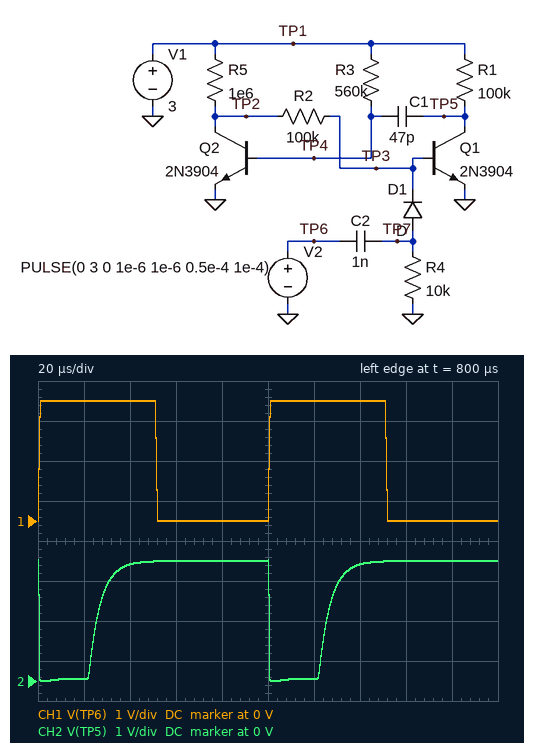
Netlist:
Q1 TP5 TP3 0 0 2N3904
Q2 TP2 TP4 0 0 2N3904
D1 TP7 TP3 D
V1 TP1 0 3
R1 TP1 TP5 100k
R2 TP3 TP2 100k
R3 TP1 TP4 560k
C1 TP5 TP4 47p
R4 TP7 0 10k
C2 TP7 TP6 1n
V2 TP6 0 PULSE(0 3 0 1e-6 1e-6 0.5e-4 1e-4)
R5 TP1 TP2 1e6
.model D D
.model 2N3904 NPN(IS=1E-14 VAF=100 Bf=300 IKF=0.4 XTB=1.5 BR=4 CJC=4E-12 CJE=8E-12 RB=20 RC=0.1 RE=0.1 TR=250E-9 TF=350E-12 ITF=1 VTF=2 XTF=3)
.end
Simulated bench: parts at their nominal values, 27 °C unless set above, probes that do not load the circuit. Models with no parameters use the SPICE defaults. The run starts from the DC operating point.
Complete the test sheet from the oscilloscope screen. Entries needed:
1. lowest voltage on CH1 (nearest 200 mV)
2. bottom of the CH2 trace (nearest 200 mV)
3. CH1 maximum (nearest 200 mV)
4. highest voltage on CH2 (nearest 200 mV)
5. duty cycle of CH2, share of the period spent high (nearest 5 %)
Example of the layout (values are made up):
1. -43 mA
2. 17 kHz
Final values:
1. 0 V
2. 0 V
3. 3.0 V
4. 3.0 V
5. 75 %
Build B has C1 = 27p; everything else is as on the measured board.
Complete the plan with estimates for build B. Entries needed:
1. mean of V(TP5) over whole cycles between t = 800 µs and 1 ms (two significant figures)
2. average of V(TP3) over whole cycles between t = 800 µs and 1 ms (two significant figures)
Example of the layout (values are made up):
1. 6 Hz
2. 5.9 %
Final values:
1. 2.5 V
2. 100 mV
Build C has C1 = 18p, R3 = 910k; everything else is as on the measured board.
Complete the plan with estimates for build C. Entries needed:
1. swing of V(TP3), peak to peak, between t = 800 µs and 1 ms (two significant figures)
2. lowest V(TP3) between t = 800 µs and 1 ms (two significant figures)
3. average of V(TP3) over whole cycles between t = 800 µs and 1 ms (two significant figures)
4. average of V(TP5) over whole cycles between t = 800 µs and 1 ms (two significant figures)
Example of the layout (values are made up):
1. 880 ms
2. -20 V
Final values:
1. 750 mV
2. 11 mV
3. 110 mV
4. 2.5 V
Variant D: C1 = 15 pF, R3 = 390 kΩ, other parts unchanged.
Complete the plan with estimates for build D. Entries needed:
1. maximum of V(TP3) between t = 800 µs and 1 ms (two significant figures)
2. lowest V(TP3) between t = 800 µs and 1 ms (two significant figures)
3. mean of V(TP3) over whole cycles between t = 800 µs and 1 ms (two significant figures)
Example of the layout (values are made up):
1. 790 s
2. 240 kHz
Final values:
1. 760 mV
2. 8.2 mV
3. 65 mV
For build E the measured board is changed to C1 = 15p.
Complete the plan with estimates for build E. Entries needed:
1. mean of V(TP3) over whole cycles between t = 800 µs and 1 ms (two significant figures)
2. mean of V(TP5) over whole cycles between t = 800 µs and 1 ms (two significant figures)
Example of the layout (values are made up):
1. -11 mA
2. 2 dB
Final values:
1. 73 mV
2. 2.7 V
